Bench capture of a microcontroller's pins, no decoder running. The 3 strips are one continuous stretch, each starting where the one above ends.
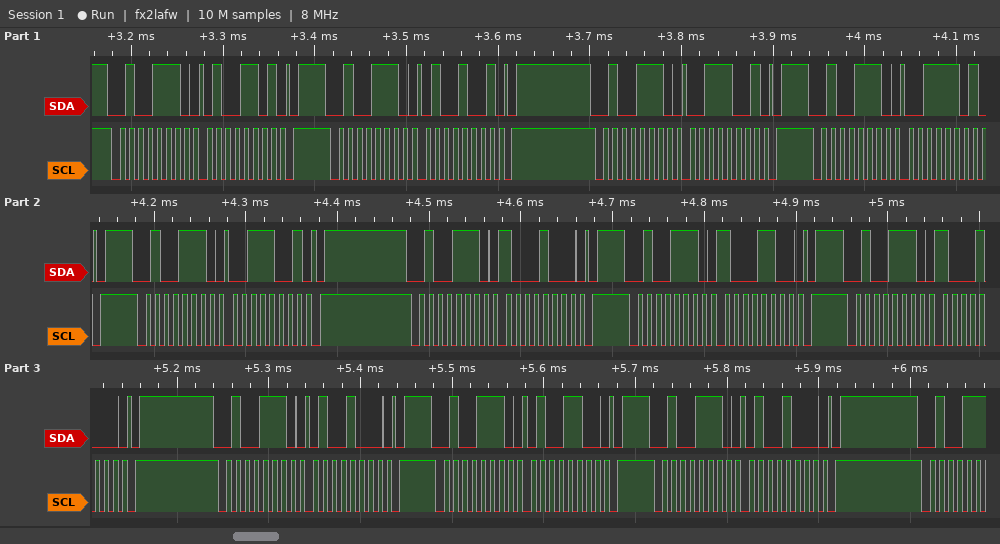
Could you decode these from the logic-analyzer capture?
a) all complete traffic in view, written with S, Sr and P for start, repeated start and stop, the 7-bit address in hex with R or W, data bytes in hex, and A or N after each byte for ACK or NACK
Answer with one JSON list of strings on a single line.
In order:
["S 27W A 4D A P S 27W A 49 A P S 27W A 39 A P S 27W A 3D A P S 27W A 39 A P S 27W A 88 A P S 27W A 8C A P S 27W A 88 A P S 27W A 48 A P S 27W A 4C A P S 27W A 48 A P"]
